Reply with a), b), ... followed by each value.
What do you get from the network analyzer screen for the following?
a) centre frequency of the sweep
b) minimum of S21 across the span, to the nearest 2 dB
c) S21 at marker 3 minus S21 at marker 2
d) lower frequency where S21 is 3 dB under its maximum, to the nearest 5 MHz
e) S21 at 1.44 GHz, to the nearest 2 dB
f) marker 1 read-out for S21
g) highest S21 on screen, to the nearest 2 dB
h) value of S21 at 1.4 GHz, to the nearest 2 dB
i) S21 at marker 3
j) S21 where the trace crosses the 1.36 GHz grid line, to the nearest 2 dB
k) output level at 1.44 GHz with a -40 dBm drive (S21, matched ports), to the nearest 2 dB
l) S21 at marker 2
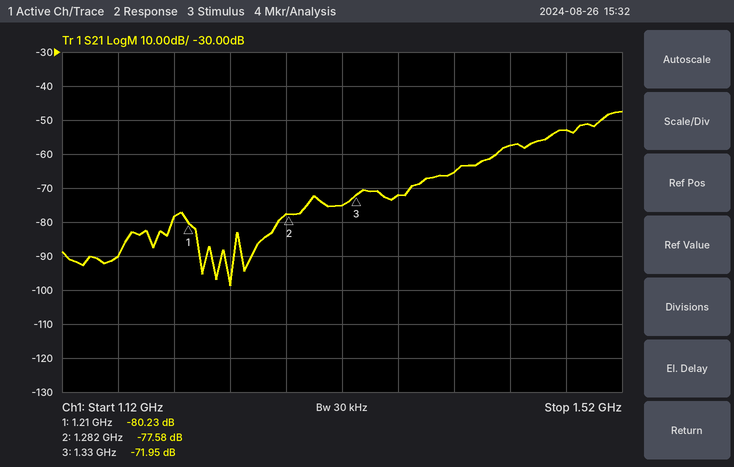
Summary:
a) 1.32 GHz
b) -98 dB
c) 5.63 dB
d) 1.505 GHz
e) -58 dB
f) -80.23 dB
g) -48 dB
h) -66 dB
i) -71.95 dB
j) -72 dB
k) -98 dBm
l) -77.58 dB
